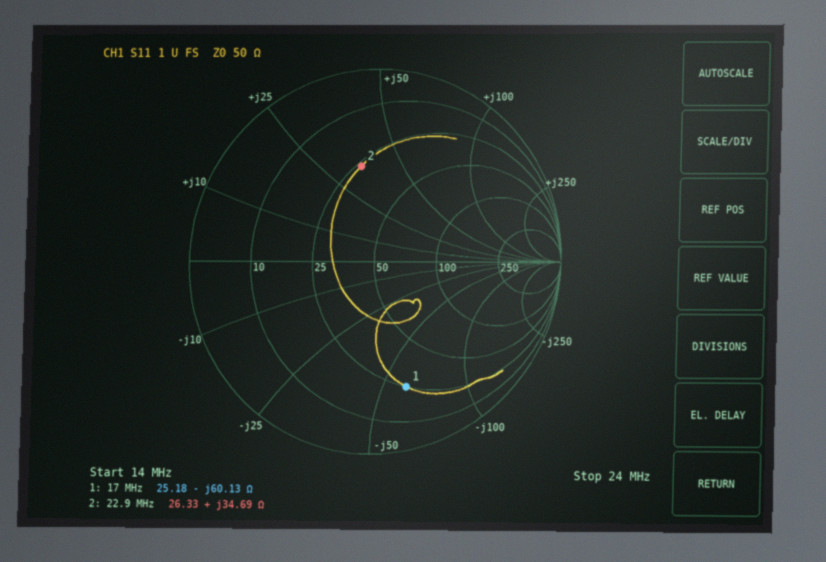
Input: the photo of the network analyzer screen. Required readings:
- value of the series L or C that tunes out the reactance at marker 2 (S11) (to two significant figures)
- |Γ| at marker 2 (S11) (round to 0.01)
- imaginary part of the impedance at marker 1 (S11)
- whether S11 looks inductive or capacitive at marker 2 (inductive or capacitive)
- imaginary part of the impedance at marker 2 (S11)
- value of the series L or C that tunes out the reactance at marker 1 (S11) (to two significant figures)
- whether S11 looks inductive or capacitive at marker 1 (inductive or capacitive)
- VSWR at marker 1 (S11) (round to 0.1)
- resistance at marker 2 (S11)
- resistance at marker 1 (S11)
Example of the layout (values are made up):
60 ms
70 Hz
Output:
200 pF
0.50
-60.13 Ω
inductive
+34.69 Ω
560 nH
capacitive
5.2
26.33 Ω
25.18 Ω
